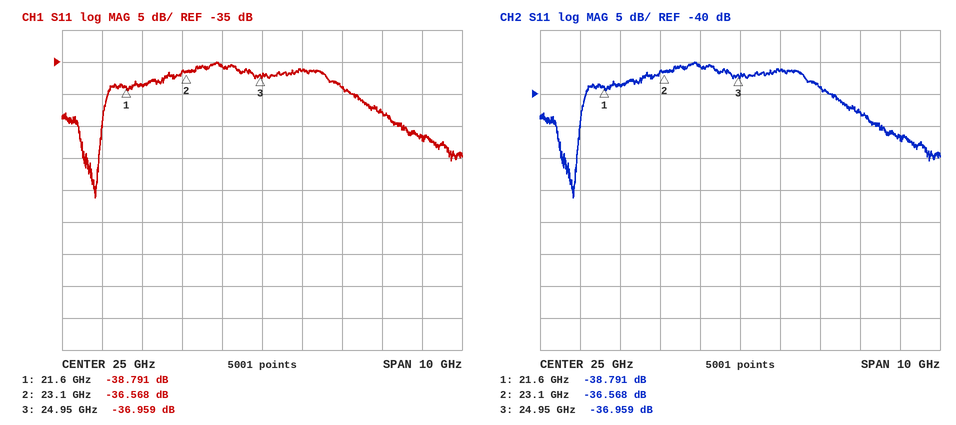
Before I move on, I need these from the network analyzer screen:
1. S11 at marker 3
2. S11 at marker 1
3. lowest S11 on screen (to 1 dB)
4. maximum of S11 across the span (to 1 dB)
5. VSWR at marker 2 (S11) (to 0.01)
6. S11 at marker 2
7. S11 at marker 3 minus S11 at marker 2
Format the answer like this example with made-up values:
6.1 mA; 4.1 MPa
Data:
-36.959 dB; -38.791 dB; -56 dB; -35 dB; 1.03; -36.568 dB; -0.391 dB
